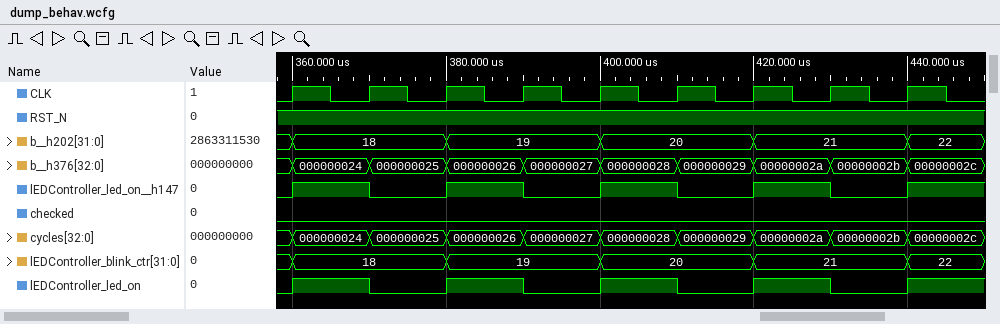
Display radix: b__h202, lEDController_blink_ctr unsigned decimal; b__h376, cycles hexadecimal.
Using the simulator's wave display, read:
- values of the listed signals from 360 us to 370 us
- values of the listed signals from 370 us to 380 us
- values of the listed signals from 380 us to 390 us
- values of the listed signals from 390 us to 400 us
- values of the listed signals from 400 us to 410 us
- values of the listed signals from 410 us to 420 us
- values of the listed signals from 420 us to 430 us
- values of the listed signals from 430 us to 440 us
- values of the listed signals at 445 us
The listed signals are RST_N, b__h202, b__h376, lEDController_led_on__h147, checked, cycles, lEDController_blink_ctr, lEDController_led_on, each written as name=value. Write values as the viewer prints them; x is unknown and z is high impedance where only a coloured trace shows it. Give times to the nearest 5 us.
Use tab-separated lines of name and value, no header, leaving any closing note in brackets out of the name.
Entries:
values of the listed signals from 360 us to 370 us	RST_N=1, b__h202=18, b__h376=000000024, lEDController_led_on__h147=1, checked=0, cycles=000000024, lEDController_blink_ctr=18, lEDController_led_on=1
values of the listed signals from 370 us to 380 us	RST_N=1, b__h202=18, b__h376=000000025, lEDController_led_on__h147=0, checked=0, cycles=000000025, lEDController_blink_ctr=18, lEDController_led_on=0
values of the listed signals from 380 us to 390 us	RST_N=1, b__h202=19, b__h376=000000026, lEDController_led_on__h147=1, checked=0, cycles=000000026, lEDController_blink_ctr=19, lEDController_led_on=1
values of the listed signals from 390 us to 400 us	RST_N=1, b__h202=19, b__h376=000000027, lEDController_led_on__h147=0, checked=0, cycles=000000027, lEDController_blink_ctr=19, lEDController_led_on=0
values of the listed signals from 400 us to 410 us	RST_N=1, b__h202=20, b__h376=000000028, lEDController_led_on__h147=1, checked=0, cycles=000000028, lEDController_blink_ctr=20, lEDController_led_on=1
values of the listed signals from 410 us to 420 us	RST_N=1, b__h202=20, b__h376=000000029, lEDController_led_on__h147=0, checked=0, cycles=000000029, lEDController_blink_ctr=20, lEDController_led_on=0
values of the listed signals from 420 us to 430 us	RST_N=1, b__h202=21, b__h376=00000002a, lEDController_led_on__h147=1, checked=0, cycles=00000002a, lEDController_blink_ctr=21, lEDController_led_on=1
values of the listed signals from 430 us to 440 us	RST_N=1, b__h202=21, b__h376=00000002b, lEDController_led_on__h147=0, checked=0, cycles=00000002b, lEDController_blink_ctr=21, lEDController_led_on=0
values of the listed signals at 445 us	RST_N=1, b__h202=22, b__h376=00000002c, lEDController_led_on__h147=1, checked=0, cycles=00000002c, lEDController_blink_ctr=22, lEDController_led_on=1
